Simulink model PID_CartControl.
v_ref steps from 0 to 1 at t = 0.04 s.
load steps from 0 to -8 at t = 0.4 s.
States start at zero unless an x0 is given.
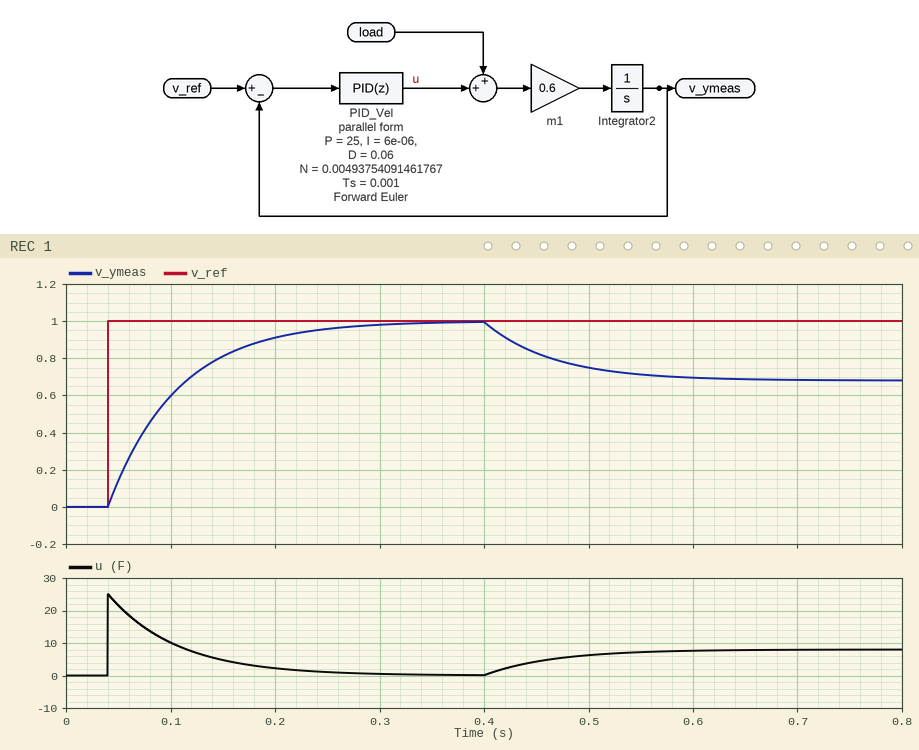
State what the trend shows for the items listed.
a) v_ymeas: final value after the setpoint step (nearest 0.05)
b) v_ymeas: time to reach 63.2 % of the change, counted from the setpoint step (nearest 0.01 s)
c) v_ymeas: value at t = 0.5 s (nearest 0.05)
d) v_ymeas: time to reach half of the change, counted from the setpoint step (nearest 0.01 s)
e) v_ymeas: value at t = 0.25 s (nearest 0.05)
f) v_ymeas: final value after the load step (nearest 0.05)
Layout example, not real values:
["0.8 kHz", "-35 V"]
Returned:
["1.00", "0.07 s", "0.75", "0.05 s", "0.95", "0.70"]
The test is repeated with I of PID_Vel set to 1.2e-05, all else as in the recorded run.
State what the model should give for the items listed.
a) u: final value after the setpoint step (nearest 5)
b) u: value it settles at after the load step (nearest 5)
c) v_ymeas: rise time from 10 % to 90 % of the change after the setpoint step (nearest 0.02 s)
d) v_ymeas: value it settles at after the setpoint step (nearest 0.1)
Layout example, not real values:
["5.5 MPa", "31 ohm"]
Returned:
["0", "10", "0.14 s", "1.0"]
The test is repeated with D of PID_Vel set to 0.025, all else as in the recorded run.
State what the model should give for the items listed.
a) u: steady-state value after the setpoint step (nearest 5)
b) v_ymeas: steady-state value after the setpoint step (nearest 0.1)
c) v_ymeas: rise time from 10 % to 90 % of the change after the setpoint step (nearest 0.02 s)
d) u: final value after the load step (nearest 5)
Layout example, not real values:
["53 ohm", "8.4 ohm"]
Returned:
["0", "1.0", "0.14 s", "10"]
